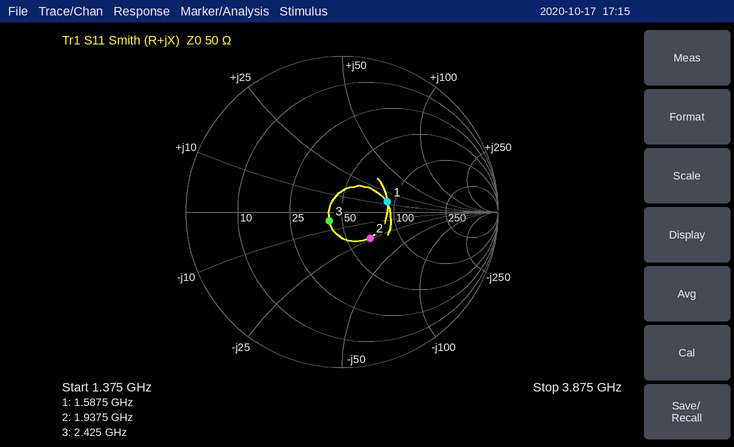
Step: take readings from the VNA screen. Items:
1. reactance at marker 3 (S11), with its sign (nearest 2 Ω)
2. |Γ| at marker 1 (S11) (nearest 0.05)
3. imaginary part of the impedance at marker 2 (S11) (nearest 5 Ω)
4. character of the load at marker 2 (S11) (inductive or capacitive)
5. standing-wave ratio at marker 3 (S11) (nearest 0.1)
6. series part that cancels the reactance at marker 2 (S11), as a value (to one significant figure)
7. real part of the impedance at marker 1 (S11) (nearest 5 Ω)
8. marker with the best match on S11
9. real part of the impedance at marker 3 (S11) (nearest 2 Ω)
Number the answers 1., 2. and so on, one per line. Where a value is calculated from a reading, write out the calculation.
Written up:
1. -4 Ω
2. 0.30
3. -25 Ω
4. capacitive
5. 1.2
6. L = 25 Ω/(2π × 1.9375 GHz) ≈ 2 nH
7. 90 Ω
8. marker 3
9. 42 Ω
